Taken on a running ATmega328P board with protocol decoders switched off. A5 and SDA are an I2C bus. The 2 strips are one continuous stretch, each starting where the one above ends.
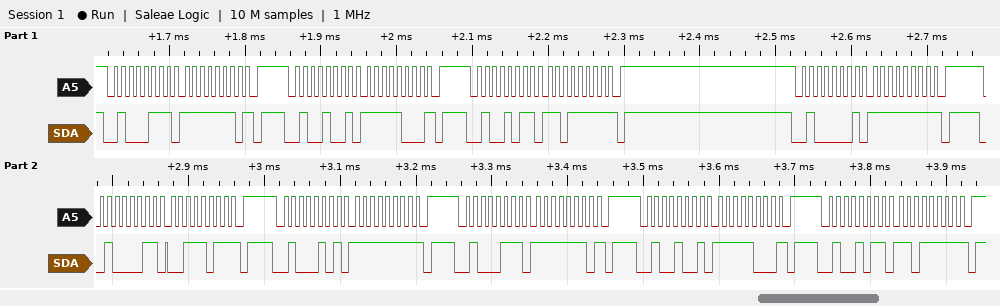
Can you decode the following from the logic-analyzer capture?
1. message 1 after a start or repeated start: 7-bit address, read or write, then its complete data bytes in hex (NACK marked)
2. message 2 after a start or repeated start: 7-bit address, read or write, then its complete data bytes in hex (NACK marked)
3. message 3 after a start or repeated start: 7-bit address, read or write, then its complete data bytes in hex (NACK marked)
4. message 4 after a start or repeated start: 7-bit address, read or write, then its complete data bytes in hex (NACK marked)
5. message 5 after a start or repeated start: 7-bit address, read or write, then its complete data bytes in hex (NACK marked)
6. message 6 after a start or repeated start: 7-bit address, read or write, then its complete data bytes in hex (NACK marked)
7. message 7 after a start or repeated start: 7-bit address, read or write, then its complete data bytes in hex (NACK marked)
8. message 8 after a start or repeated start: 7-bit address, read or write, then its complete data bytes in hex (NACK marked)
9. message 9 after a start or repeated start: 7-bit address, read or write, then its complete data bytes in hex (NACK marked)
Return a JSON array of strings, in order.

["0x23 read: FE NACK", "0x24 read: F8 NACK", "0x25 read: DF NACK", "0x20 read: FF NACK", "0x21 read: 3B NACK", "0x22 read: FF NACK", "0x23 read: FE NACK", "0x24 read: F8 NACK", "0x25 read: DF NACK"]
